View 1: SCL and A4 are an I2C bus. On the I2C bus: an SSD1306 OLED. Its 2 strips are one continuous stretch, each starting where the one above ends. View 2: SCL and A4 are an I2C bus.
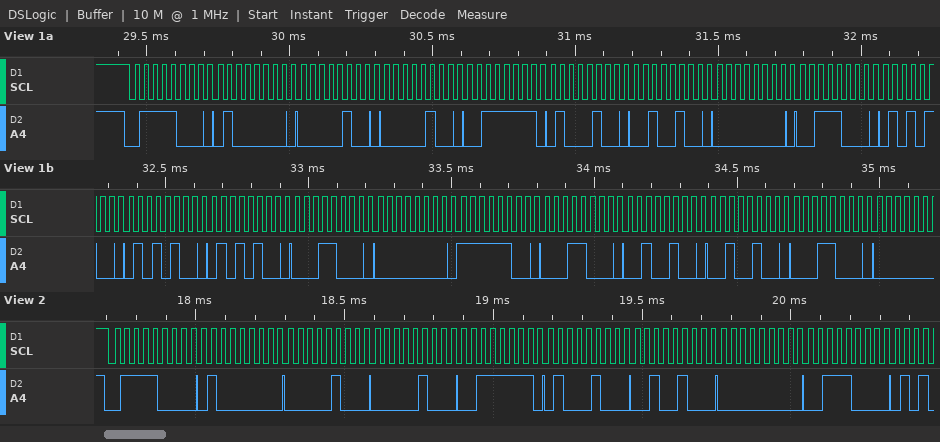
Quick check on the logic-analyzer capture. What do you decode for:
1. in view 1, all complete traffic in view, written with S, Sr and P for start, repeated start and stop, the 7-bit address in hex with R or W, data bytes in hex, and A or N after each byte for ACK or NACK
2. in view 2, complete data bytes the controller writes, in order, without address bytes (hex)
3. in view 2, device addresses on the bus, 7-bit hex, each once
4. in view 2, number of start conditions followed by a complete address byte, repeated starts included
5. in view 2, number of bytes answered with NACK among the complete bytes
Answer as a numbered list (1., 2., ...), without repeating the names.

1. S 3CW A 40 A 04 A 04 A 3F A 44 A 24 A 00 A 38 A 54 A 54 A 54 A 18 A 00 A FC A 18 A 24 A 24 A 18 A
2. 40 04 04 3F 44 24 00 38
3. 0x3C
4. 1
5. 0
